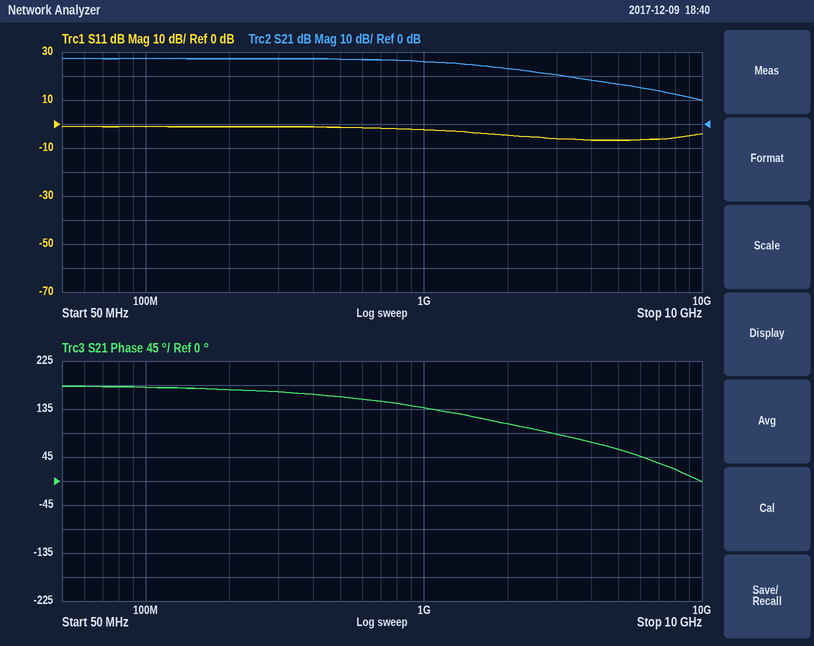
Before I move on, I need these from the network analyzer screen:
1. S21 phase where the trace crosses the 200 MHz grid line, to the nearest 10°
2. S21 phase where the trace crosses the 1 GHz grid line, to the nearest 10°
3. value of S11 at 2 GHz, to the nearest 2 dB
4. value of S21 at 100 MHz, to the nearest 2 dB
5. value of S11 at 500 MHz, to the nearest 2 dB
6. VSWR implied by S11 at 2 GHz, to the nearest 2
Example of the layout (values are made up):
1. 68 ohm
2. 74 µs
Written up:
1. 170°
2. 140°
3. -4 dB
4. 28 dB
5. -2 dB
6. 4
